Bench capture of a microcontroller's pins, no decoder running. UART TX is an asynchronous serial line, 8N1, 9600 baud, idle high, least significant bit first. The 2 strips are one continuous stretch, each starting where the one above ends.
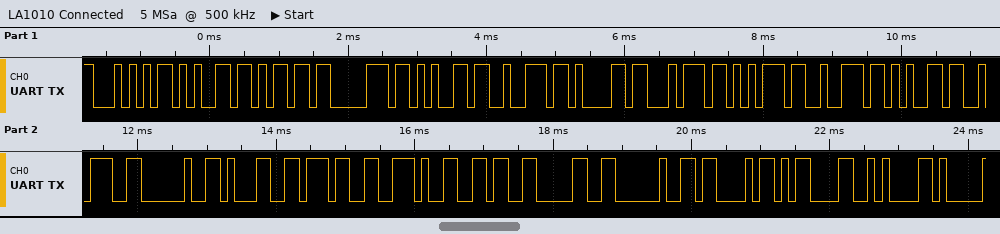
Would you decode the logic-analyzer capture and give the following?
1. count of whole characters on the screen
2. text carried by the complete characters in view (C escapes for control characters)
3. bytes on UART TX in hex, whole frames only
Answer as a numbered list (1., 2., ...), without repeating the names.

1. 22
2. "Temperature: 17.60 C\r\n"
3. 54 65 6D 70 65 72 61 74 75 72 65 3A 20 31 37 2E 36 30 20 43 0D 0A
